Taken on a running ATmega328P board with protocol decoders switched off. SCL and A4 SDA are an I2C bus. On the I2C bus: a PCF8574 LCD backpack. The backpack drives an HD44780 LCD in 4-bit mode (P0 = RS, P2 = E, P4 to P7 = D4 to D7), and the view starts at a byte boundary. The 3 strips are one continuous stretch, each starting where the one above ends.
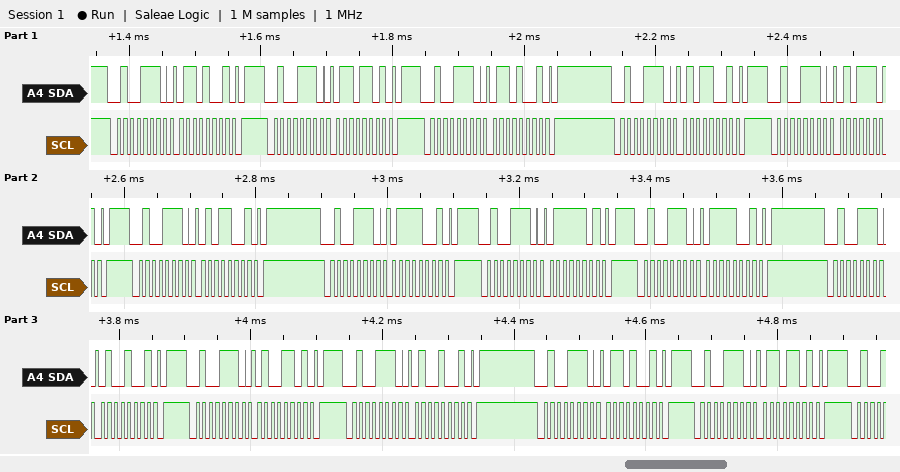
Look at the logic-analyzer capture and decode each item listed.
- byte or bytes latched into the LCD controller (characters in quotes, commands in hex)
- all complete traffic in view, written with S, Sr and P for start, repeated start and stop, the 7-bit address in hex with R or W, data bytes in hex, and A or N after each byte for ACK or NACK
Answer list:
'e' 't'
S 27W A 69 A P S 27W A 6D A P S 27W A 69 A P S 27W A 59 A P S 27W A 5D A P S 27W A 59 A P S 27W A 79 A P S 27W A 7D A P S 27W A 79 A P S 27W A 49 A P S 27W A 4D A P S 27W A 49 A P S 27W A 69 A P S 27W A 6D A P
